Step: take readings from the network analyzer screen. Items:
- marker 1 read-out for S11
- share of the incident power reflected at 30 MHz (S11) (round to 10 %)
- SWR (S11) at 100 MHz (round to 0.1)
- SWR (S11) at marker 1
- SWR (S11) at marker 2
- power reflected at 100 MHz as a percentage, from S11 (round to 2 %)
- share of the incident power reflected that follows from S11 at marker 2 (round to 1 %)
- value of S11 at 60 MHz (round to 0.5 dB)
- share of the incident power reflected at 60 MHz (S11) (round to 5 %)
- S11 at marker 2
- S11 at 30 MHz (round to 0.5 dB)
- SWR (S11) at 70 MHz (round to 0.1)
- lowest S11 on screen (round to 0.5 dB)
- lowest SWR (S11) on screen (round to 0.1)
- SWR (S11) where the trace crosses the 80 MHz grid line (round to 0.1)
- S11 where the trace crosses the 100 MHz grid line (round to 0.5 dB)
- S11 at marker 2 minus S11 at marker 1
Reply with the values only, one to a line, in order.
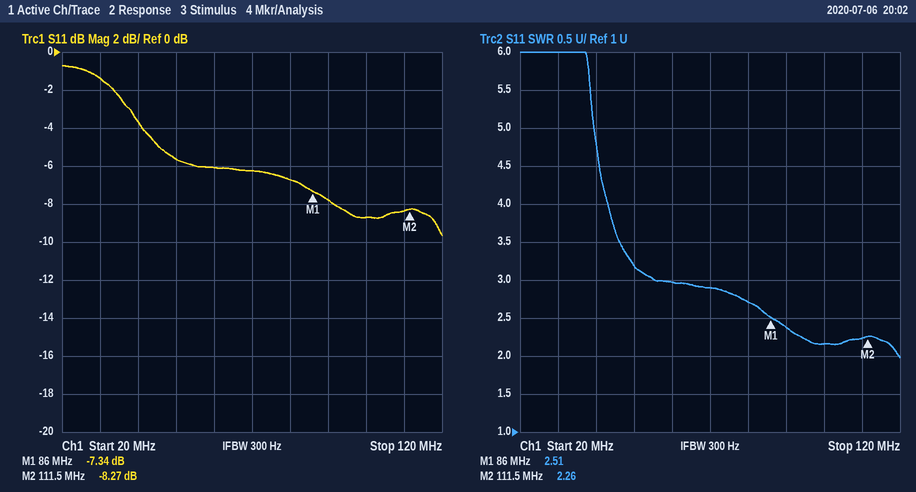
-7.34 dB
70 %
2.2
2.51
2.26
14 %
15 %
-6.0 dB
25 %
-8.27 dB
-1.5 dB
2.9
-9.5 dB
2.0
2.7
-8.5 dB
-0.93 dB
